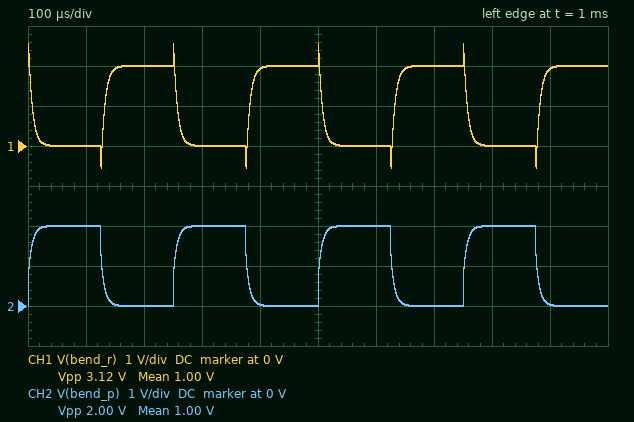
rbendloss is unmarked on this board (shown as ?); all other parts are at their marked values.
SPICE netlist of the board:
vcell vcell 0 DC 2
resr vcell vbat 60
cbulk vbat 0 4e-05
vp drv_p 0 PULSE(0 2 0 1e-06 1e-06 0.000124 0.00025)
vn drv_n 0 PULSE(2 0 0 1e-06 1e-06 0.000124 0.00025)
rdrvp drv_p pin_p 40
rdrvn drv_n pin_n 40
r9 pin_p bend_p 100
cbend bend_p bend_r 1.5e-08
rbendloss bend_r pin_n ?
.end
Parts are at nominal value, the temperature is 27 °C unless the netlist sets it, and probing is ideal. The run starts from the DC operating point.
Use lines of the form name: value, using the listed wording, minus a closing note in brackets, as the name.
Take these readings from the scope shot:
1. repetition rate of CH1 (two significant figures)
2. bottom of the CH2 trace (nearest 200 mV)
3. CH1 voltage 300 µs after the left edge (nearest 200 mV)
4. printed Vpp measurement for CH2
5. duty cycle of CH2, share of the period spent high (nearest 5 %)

repetition rate of CH1: 4.0 kHz
bottom of the CH2 trace: 0 V
CH1 voltage 300 µs after the left edge: 0 V
printed Vpp measurement for CH2: 2.00 V
duty cycle of CH2, share of the period spent high: 50 %
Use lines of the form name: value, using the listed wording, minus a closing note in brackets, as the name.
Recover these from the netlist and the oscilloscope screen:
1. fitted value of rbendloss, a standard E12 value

fitted value of rbendloss, a standard E12 value: 270 Ω
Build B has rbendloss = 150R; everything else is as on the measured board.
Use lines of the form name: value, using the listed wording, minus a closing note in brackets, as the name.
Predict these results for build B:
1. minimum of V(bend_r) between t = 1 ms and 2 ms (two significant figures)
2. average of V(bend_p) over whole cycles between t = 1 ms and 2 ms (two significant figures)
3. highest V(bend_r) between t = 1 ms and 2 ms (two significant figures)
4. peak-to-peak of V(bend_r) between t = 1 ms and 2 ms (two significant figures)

minimum of V(bend_r) between t = 1 ms and 2 ms: -100 mV
average of V(bend_p) over whole cycles between t = 1 ms and 2 ms: 1.0 V
highest V(bend_r) between t = 1 ms and 2 ms: 2.1 V
peak-to-peak of V(bend_r) between t = 1 ms and 2 ms: 2.2 V
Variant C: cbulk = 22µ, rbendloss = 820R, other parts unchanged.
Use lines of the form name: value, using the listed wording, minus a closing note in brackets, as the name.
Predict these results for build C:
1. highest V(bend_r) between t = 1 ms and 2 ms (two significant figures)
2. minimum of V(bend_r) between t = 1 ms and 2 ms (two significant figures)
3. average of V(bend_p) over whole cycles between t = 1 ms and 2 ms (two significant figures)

highest V(bend_r) between t = 1 ms and 2 ms: 3.3 V
minimum of V(bend_r) between t = 1 ms and 2 ms: -1.3 V
average of V(bend_p) over whole cycles between t = 1 ms and 2 ms: 1.0 V
